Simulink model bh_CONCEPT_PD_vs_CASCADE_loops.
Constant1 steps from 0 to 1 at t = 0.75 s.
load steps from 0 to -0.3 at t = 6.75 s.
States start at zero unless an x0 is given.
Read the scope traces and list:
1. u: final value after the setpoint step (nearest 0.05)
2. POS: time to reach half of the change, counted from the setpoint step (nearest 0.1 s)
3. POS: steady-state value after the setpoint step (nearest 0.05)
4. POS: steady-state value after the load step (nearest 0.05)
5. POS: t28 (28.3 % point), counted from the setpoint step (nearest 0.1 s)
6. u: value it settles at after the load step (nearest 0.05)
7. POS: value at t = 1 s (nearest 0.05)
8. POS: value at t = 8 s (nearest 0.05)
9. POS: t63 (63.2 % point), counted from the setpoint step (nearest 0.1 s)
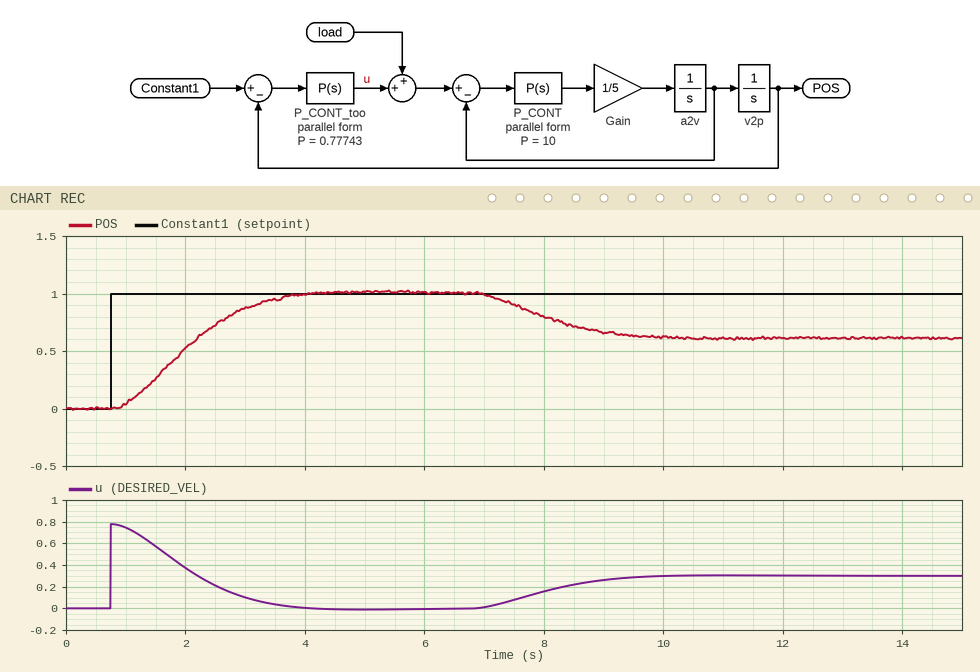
0.00
1.2 s
1.00
0.60
0.8 s
0.30
0.05
0.80
1.5 s
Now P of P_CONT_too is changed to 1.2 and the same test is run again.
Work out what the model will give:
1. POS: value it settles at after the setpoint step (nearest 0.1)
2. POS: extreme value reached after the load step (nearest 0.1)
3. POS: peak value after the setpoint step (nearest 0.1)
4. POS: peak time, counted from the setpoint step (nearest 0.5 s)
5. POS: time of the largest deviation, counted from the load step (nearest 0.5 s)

1.0
0.7
1.1
2.5 s
2.5 s
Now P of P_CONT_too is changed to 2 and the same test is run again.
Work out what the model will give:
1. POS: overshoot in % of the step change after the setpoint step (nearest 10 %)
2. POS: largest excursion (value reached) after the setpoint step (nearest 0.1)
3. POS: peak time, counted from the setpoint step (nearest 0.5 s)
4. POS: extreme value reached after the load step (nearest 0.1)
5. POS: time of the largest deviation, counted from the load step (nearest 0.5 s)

20 %
1.2
2.0 s
0.8
2.0 s
